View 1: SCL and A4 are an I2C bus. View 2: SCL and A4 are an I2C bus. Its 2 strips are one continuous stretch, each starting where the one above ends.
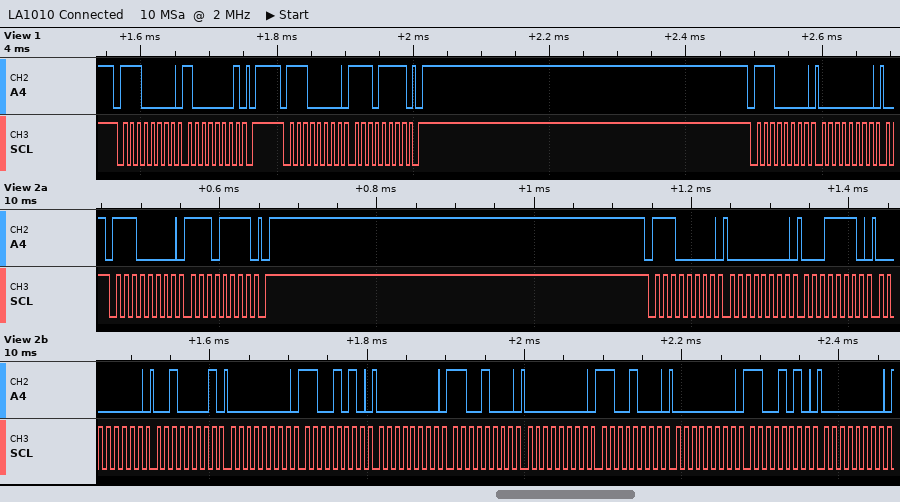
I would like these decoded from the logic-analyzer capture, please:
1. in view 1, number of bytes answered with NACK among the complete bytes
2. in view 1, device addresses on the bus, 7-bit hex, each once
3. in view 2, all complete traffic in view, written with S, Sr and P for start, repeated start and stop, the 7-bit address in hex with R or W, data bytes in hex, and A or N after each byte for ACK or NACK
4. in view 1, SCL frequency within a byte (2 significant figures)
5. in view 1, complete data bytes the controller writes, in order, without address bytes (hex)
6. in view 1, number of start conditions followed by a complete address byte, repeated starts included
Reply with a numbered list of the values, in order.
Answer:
1. 0
2. 0x70
3. S 70W A EF A P S 70W A 00 A 1E A 00 A 21 A 00 A CA A 00 A C8 A 00 A C8 A 00 A CA A 00 A
4. 100 kHz
5. 81 EF 00
6. 3
